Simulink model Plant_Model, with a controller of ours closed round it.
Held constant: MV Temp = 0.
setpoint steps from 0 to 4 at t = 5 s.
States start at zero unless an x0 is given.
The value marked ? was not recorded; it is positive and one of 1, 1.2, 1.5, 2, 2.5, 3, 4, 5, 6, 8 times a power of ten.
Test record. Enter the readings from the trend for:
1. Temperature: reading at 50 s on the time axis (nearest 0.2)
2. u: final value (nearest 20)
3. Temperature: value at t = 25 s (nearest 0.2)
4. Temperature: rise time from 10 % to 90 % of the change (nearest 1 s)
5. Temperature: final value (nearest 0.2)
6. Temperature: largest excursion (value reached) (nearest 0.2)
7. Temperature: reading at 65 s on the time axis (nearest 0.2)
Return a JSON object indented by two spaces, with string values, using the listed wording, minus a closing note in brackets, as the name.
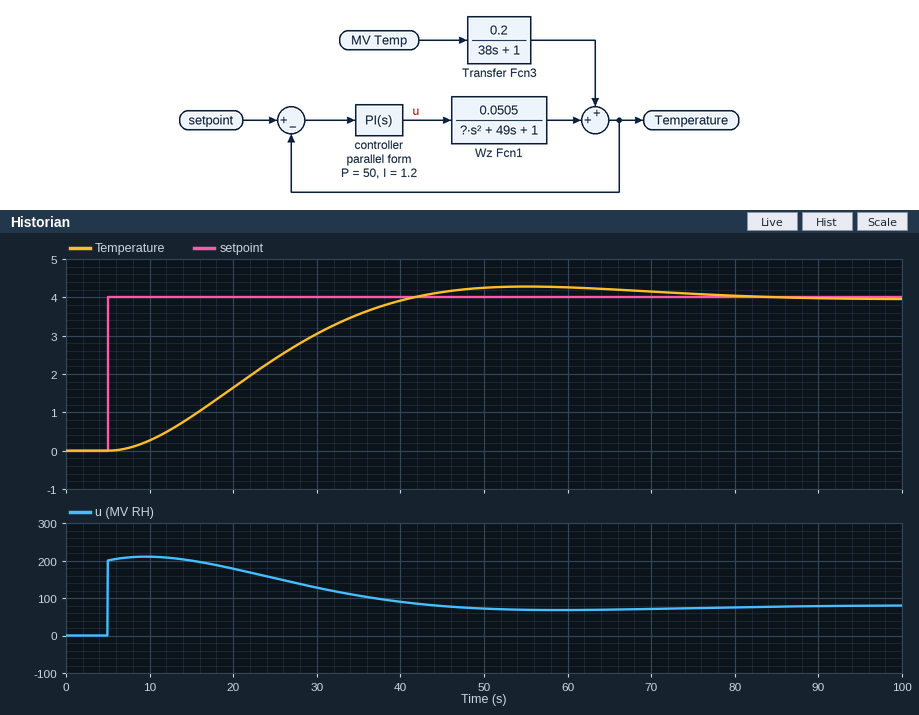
{
  "Temperature: reading at 50 s on the time axis": "4.2",
  "u: final value": "80",
  "Temperature: value at t = 25 s": "2.4",
  "Temperature: rise time from 10 % to 90 % of the change": "24 s",
  "Temperature: final value": "4.0",
  "Temperature: largest excursion (value reached)": "4.2",
  "Temperature: reading at 65 s on the time axis": "4.2"
}
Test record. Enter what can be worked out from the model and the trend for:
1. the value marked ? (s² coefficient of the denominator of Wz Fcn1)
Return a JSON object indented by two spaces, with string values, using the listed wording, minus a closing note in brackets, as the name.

{
  "the value marked ?": "400"
}
